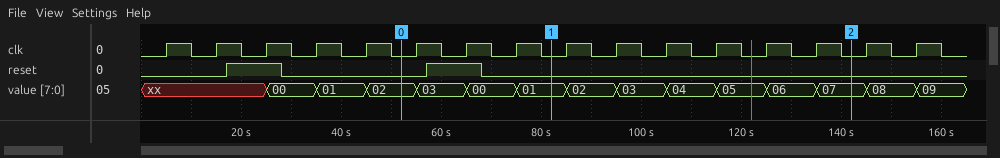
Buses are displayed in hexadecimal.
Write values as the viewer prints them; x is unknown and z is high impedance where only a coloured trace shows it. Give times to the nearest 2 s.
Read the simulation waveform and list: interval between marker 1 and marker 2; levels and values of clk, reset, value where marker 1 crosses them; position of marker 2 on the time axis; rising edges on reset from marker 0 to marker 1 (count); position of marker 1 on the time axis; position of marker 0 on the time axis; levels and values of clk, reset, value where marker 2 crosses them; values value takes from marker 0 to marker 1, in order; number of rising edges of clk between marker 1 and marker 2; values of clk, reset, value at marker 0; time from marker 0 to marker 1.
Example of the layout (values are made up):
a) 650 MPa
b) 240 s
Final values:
a) 60 s
b) clk=0, reset=0, value=01
c) 142 s
d) 1
e) 82 s
f) 52 s
g) clk=0, reset=0, value=07
h) 02, 03, 00, 01
i) 6
j) clk=0, reset=0, value=02
k) 30 s
